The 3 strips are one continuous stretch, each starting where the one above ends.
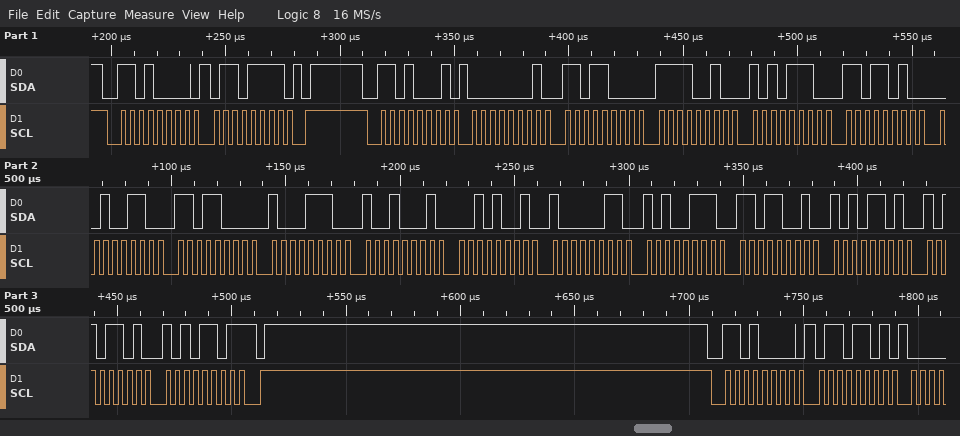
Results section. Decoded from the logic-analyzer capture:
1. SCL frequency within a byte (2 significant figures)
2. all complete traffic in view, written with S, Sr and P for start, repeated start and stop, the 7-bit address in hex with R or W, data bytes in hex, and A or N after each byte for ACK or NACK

250 kHz
S 68W A 6F A P S 68R A 01 A D8 A F2 A AE A DA A 26 A D8 A 8E A 91 A 29 A 83 A A7 A D9 A AD A AD A AD N P S 68W A 6D A
